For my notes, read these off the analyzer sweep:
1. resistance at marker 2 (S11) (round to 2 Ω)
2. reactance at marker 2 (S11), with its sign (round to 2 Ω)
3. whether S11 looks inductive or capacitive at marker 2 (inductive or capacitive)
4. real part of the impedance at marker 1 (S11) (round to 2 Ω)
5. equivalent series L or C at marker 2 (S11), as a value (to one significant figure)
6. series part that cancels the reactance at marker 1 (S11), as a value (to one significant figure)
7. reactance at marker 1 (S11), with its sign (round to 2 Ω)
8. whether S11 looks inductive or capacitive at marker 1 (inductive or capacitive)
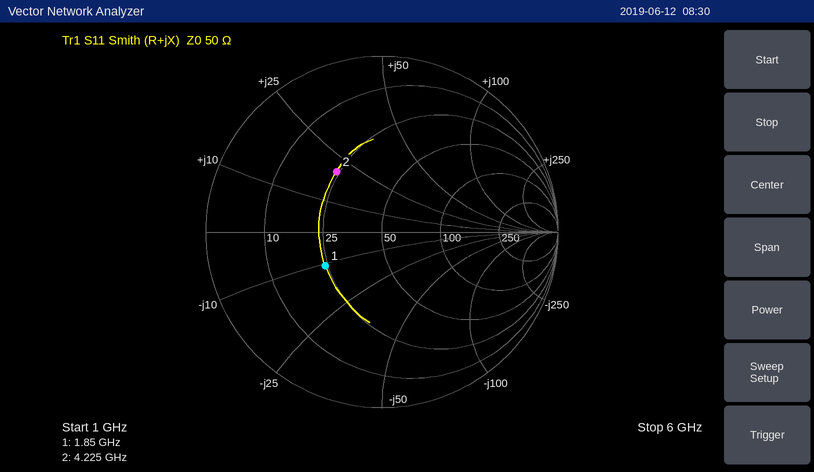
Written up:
24 Ω
+20 Ω
inductive
24 Ω
800 pH
900 pH
-10 Ω
capacitive
